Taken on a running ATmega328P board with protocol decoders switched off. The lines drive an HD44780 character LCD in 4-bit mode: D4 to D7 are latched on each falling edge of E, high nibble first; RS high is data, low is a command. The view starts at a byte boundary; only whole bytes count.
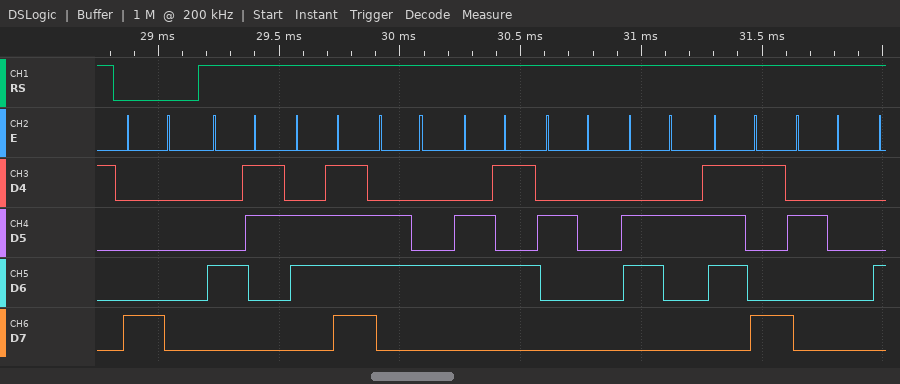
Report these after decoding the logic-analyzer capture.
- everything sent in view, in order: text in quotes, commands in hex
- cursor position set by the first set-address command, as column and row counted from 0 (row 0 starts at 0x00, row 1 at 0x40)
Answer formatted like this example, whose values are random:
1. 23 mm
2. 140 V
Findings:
1. 0x80 "Code by "
2. column 0, row 0
